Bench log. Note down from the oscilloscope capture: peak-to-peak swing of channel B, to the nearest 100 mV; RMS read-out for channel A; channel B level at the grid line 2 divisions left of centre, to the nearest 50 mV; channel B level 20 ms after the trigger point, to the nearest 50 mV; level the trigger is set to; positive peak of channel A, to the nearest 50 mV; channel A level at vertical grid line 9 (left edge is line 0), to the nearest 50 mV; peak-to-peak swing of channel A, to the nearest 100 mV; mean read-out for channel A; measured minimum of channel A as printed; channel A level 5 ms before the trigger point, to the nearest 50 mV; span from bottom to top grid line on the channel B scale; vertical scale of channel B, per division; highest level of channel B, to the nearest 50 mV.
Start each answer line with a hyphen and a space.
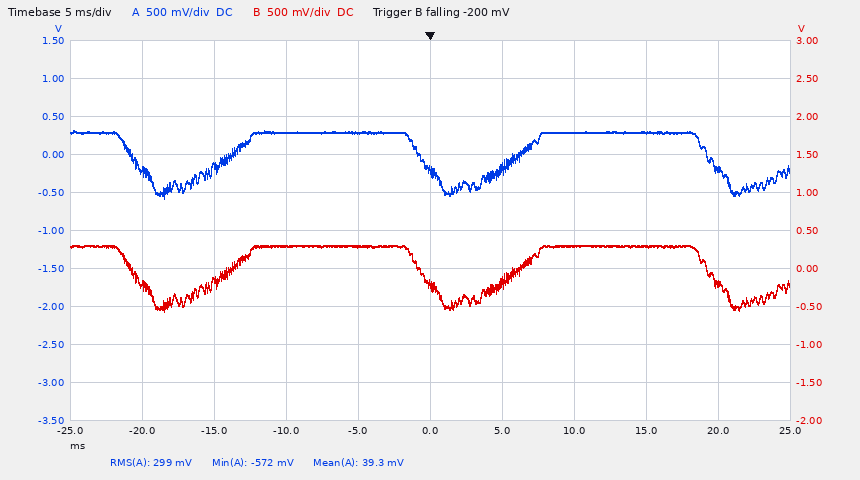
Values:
- 900 mV
- 299 mV
- 300 mV
- -200 mV
- -200 mV
- 300 mV
- -200 mV
- 900 mV
- 39.3 mV
- -572 mV
- 300 mV
- 5 V
- 500 mV
- 300 mV
